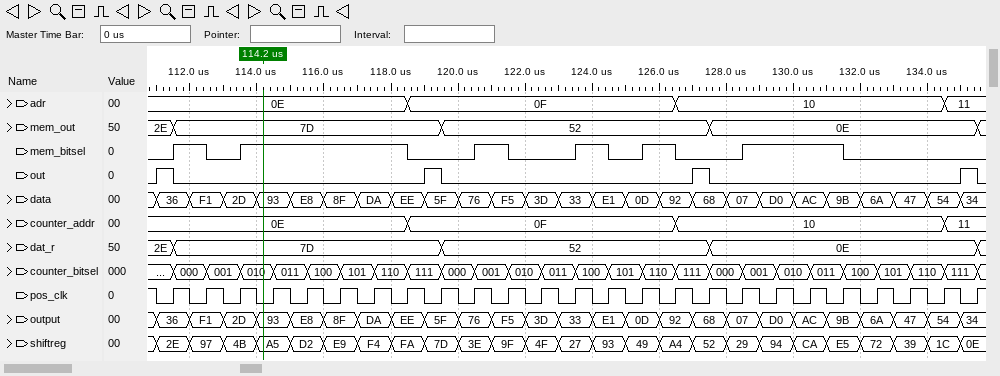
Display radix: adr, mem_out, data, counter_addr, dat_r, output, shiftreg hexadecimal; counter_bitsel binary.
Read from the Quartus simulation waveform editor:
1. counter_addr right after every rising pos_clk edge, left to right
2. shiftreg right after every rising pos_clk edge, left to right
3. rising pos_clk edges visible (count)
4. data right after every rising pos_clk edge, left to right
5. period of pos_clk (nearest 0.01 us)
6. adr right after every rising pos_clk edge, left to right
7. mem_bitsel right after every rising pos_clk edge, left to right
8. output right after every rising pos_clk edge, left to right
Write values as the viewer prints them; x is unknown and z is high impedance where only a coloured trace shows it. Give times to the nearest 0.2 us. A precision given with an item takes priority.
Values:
0E, 0E, 0E, 0E, 0E, 0E, 0E, 0F, 0F, 0F, 0F, 0F, 0F, 0F, 0F, 10, 10, 10, 10, 10, 10, 10, 10, 11, 11
2E, 97, 4B, A5, D2, E9, F4, FA, 7D, 3E, 9F, 4F, 27, 93, 49, A4, 52, 29, 94, CA, E5, 72, 39, 1C, 0E
25
36, F1, 2D, 93, E8, 8F, DA, EE, 5F, 76, F5, 3D, 33, E1, 0D, 92, 68, 07, D0, AC, 9B, 6A, 47, 54, 34
1 us
0E, 0E, 0E, 0E, 0E, 0E, 0E, 0F, 0F, 0F, 0F, 0F, 0F, 0F, 0F, 10, 10, 10, 10, 10, 10, 10, 10, 11, 11
1 0 1 1 1 1 1 0 0 1 0 0 1 0 1 0 0 1 1 1 0 0 0 0 0
36, F1, 2D, 93, E8, 8F, DA, EE, 5F, 76, F5, 3D, 33, E1, 0D, 92, 68, 07, D0, AC, 9B, 6A, 47, 54, 34
